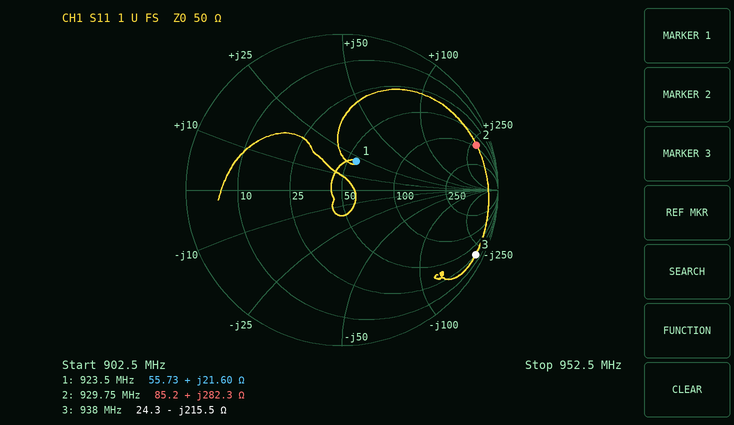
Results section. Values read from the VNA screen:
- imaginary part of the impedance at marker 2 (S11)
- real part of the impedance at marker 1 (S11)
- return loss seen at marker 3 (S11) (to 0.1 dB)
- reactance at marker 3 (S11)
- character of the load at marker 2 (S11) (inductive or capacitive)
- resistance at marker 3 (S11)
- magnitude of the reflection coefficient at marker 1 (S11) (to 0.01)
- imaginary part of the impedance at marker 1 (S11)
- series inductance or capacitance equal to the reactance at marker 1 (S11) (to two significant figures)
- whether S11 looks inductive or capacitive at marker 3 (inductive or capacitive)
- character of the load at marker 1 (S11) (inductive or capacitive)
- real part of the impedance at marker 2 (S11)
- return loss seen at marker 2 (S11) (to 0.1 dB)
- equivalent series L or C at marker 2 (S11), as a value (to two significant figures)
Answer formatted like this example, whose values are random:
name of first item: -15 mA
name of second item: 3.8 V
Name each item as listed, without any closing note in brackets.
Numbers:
imaginary part of the impedance at marker 2: +282.3 Ω
real part of the impedance at marker 1: 55.73 Ω
return loss seen at marker 3 (S11): 0.4 dB
reactance at marker 3: -215.5 Ω
character of the load at marker 2 (S11): inductive
resistance at marker 3: 24.3 Ω
magnitude of the reflection coefficient at marker 1 (S11): 0.21
imaginary part of the impedance at marker 1: +21.60 Ω
series inductance or capacitance equal to the reactance at marker 1 (S11): 3.7 nH
whether S11 looks inductive or capacitive at marker 3: capacitive
character of the load at marker 1 (S11): inductive
real part of the impedance at marker 2: 85.2 Ω
return loss seen at marker 2 (S11): 0.8 dB
equivalent series L or C at marker 2 (S11), as a value: 48 nH
